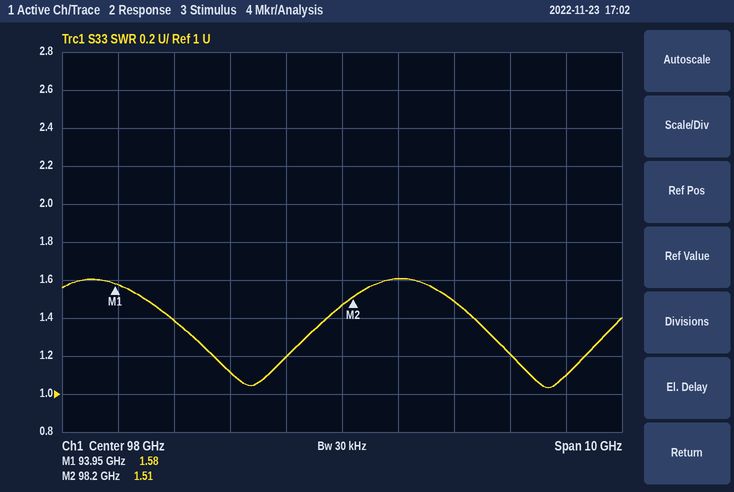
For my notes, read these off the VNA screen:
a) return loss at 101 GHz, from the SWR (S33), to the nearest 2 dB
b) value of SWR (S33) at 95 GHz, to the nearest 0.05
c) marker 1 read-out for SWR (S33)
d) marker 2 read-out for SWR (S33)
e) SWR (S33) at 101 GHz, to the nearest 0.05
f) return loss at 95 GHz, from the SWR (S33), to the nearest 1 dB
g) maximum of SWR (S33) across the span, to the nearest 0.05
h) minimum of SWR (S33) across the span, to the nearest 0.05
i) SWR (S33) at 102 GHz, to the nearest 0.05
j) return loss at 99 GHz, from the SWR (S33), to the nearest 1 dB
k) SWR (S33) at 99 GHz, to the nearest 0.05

20 dB
1.40
1.58
1.51
1.20
16 dB
1.60
1.05
1.10
13 dB
1.60
